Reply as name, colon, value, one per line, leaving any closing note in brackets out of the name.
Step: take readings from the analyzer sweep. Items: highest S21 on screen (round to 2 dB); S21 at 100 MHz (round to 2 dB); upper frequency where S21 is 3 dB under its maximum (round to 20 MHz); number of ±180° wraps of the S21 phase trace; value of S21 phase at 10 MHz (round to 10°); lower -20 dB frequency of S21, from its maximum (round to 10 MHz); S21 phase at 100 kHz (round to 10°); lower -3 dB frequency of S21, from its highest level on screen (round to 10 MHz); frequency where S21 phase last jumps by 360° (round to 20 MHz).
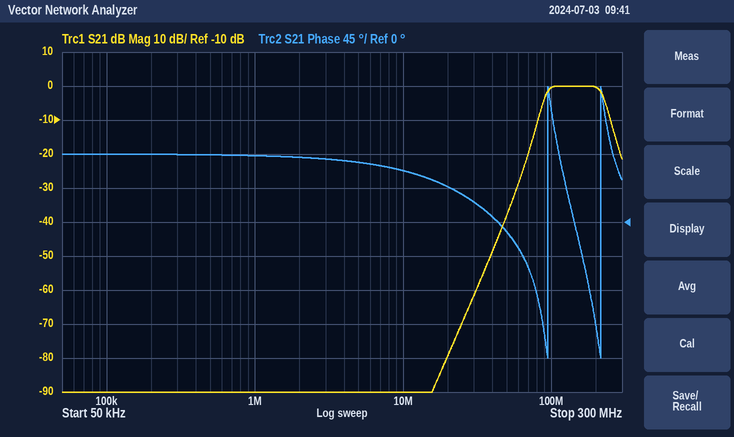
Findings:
highest S21 on screen: 0 dB
S21 at 100 MHz: 0 dB
upper frequency where S21 is 3 dB under its maximum: 220 MHz
number of ±180° wraps of the S21 phase trace: 2
value of S21 phase at 10 MHz: 70°
lower -20 dB frequency of S21, from its maximum: 70 MHz
S21 phase at 100 kHz: 90°
lower -3 dB frequency of S21, from its highest level on screen: 90 MHz
frequency where S21 phase last jumps by 360°: 220 MHz
